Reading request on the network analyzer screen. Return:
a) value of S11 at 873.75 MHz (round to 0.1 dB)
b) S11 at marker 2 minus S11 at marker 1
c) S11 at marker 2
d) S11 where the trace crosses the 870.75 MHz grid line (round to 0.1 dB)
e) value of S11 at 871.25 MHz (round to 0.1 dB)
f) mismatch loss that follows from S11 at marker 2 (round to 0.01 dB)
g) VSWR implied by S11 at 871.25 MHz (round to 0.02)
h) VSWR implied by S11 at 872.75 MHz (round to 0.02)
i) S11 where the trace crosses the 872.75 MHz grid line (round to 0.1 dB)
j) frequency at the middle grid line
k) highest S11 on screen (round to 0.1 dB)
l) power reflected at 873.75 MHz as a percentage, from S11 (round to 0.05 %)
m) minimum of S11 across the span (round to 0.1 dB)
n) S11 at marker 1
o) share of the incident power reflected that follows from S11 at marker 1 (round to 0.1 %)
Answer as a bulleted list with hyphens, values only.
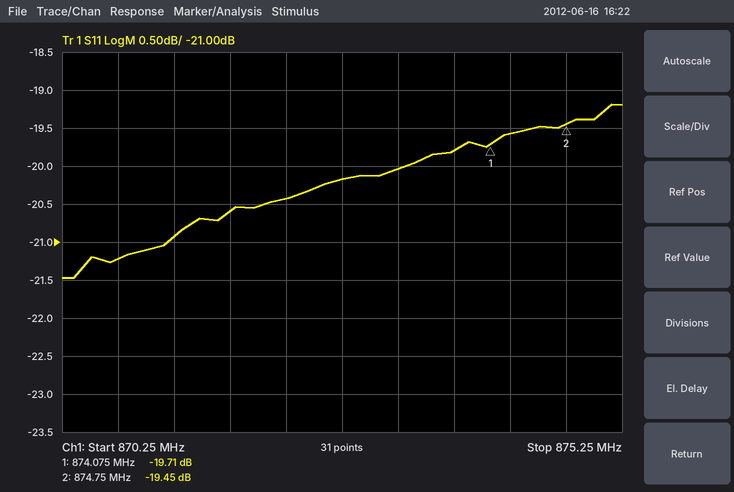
- -19.8 dB
- 0.26 dB
- -19.45 dB
- -21.2 dB
- -20.9 dB
- 0.05 dB
- 1.20
- 1.22
- -20.2 dB
- 872.75 MHz
- -19.2 dB
- 1.05 %
- -21.5 dB
- -19.71 dB
- 1.1 %
